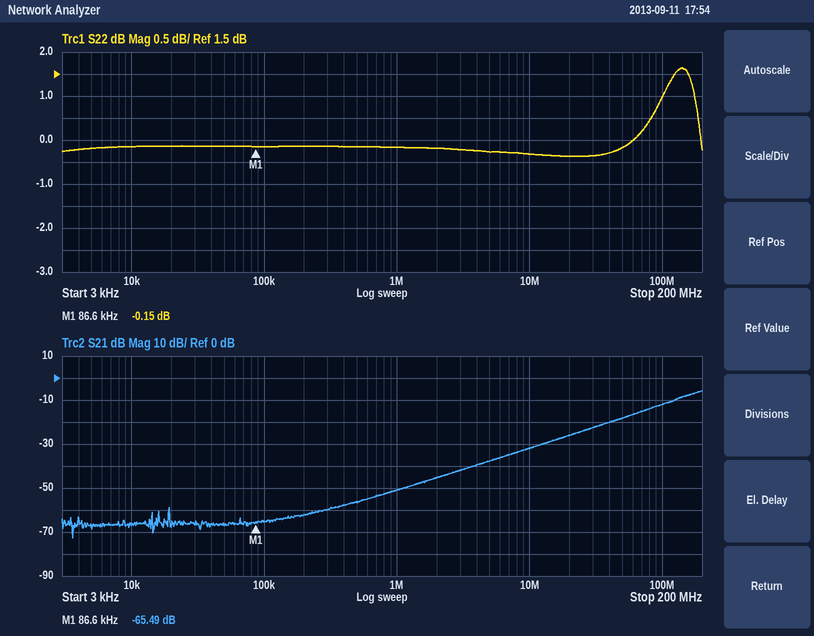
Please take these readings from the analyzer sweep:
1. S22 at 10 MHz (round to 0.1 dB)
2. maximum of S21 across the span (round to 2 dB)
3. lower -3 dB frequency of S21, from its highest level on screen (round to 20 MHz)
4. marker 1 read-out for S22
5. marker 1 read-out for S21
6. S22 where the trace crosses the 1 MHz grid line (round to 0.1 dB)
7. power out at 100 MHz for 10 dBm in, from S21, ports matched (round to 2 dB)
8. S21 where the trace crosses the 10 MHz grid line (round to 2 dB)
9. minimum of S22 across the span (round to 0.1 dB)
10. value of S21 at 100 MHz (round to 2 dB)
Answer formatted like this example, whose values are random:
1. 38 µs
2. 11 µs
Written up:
1. -0.3 dB
2. -6 dB
3. 140 MHz
4. -0.15 dB
5. -65.49 dB
6. -0.2 dB
7. -2 dBm
8. -32 dB
9. -0.4 dB
10. -12 dB
